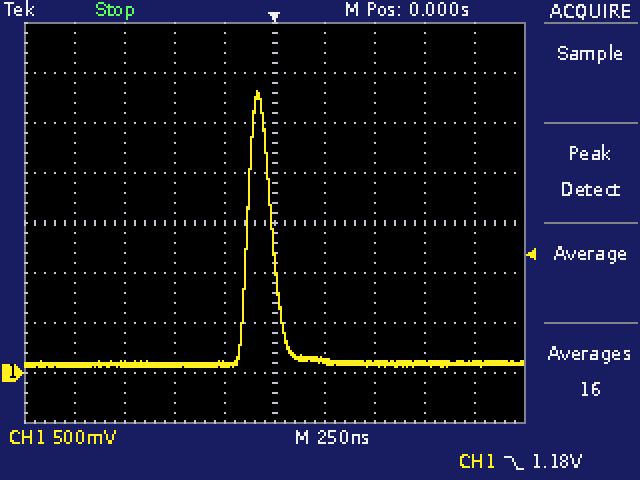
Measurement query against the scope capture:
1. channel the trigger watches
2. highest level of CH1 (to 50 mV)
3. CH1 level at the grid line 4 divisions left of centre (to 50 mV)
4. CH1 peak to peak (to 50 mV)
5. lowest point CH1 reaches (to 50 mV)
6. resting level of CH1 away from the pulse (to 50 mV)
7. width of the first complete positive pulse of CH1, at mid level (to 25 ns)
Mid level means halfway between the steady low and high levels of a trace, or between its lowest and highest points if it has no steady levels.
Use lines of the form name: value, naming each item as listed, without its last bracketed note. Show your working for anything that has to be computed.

channel the trigger watches: CH1
highest level of CH1: 2.80 V
CH1 level at the grid line 4 divisions left of centre: 100 mV
CH1 peak to peak: 2.80 V − (50 mV) = 2.75 V
lowest point CH1 reaches: 50 mV
resting level of CH1 away from the pulse: 100 mV
width of the first complete positive pulse of CH1, at mid level: 125 ns
